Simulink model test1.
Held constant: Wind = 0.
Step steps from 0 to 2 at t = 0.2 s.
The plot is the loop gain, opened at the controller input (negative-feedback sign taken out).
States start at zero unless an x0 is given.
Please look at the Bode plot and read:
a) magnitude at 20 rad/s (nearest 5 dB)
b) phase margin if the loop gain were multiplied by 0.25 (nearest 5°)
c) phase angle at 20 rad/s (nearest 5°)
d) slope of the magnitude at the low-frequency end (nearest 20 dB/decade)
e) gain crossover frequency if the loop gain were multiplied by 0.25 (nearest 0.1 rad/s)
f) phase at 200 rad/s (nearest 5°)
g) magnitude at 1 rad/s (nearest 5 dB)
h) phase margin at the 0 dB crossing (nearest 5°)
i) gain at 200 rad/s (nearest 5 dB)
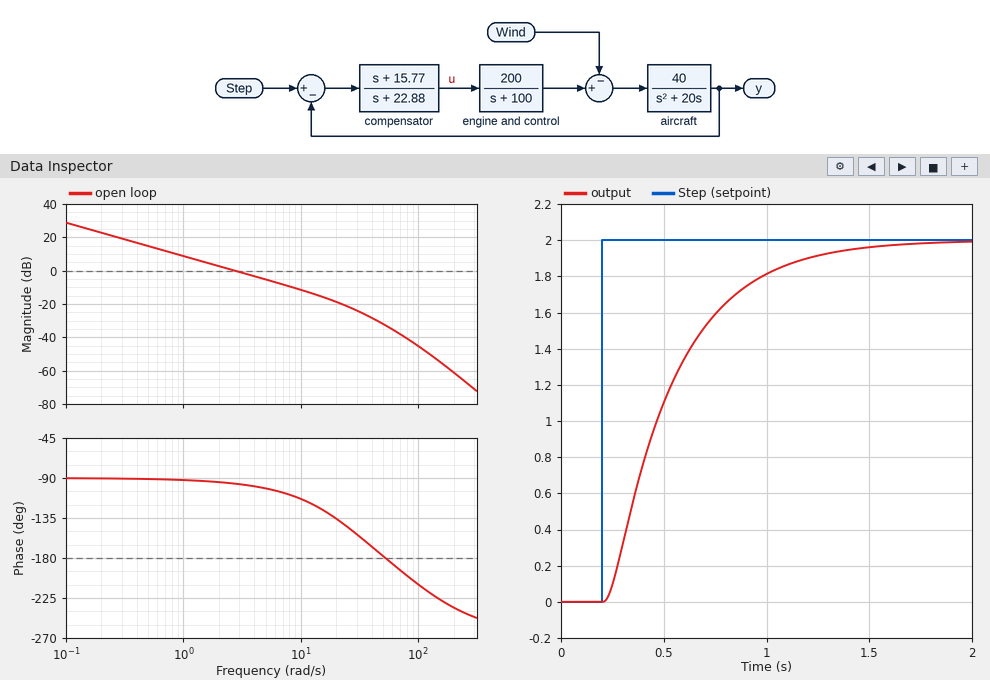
-20 dB
90°
-135°
-20 dB/decade
0.7 rad/s
-235°
10 dB
85°
-60 dB
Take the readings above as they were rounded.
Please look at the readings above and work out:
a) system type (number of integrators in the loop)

1
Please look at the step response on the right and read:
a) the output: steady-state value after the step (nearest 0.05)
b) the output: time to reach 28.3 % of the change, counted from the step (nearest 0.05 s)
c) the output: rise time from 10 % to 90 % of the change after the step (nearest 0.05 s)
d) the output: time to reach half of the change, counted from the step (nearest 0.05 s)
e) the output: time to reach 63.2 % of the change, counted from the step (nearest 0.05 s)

2.00
0.15 s
0.70 s
0.25 s
0.35 s
